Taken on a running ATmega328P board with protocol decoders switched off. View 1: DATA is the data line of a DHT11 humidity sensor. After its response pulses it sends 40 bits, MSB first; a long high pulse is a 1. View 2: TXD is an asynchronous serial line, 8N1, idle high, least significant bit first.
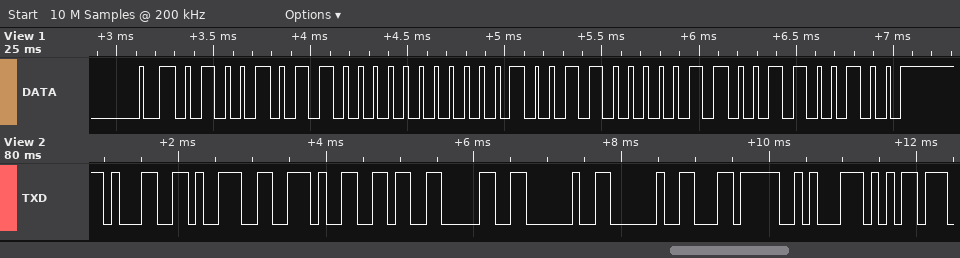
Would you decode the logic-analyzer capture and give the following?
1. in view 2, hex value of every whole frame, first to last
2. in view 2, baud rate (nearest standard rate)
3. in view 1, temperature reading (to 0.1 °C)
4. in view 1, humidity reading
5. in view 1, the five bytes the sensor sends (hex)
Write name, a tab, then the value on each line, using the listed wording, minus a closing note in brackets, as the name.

in view 2, hex value of every whole frame, first to last	31 39 2E 36 30 20 20 EC 8A B5
in view 2, baud rate	9600 baud
in view 1, temperature reading	19.6 °C
in view 1, humidity reading	75 %
in view 1, the five bytes the sensor sends	4B 00 13 06 64
